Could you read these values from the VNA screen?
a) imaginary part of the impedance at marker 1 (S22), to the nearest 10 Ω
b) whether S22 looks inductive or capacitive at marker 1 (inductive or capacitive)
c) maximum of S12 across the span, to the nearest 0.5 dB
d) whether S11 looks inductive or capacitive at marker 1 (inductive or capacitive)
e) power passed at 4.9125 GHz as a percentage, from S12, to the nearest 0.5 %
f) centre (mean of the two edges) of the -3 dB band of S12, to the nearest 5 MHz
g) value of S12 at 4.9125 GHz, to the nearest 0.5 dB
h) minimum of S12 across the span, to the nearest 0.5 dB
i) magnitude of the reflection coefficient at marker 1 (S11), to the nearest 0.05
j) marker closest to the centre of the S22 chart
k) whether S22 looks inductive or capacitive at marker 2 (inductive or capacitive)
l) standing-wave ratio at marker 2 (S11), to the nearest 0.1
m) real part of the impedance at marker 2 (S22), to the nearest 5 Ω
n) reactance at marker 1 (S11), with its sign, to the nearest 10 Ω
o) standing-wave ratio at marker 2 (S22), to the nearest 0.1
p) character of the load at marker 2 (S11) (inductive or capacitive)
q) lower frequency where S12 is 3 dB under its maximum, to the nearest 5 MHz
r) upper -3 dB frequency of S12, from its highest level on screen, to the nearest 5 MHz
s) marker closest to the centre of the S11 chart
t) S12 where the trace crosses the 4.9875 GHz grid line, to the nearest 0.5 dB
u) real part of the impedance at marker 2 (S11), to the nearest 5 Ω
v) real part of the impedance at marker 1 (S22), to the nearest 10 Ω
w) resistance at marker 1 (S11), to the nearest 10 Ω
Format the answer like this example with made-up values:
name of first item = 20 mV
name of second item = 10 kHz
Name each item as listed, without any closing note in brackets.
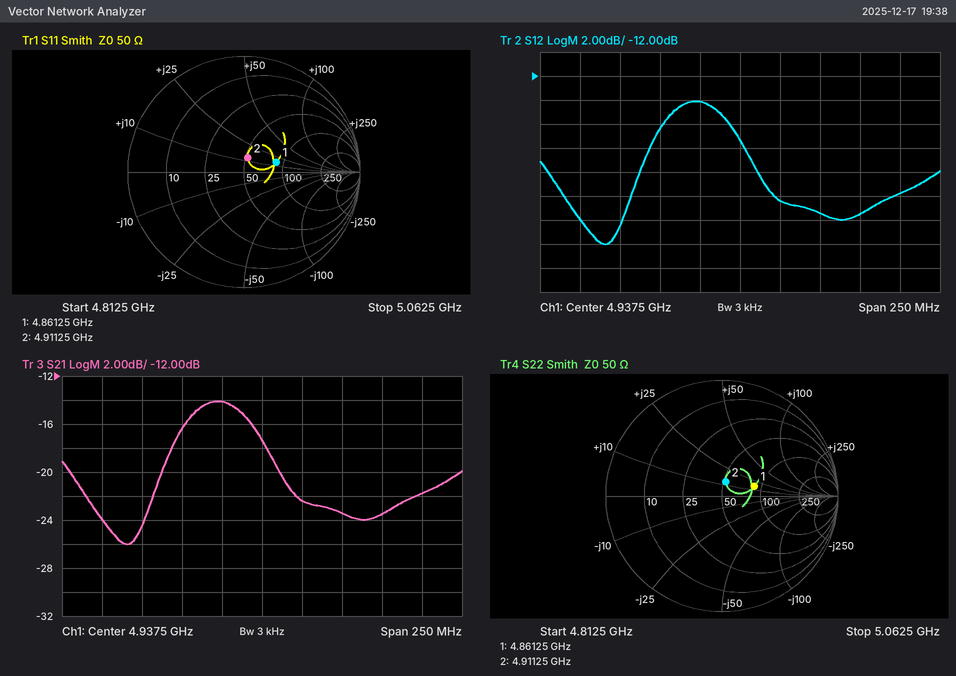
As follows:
imaginary part of the impedance at marker 1 (S22), to the nearest 10 Ω = +20 Ω
whether S22 looks inductive or capacitive at marker 1 = inductive
maximum of S12 across the span, to the nearest 0.5 dB = -14.0 dB
whether S11 looks inductive or capacitive at marker 1 = inductive
power passed at 4.9125 GHz as a percentage, from S12, to the nearest 0.5 % = 4.0 %
centre (mean of the two edges) of the -3 dB band of S12, to the nearest 5 MHz = 4.910 GHz
value of S12 at 4.9125 GHz, to the nearest 0.5 dB = -14.0 dB
minimum of S12 across the span, to the nearest 0.5 dB = -26.0 dB
magnitude of the reflection coefficient at marker 1 (S11), to the nearest 0.05 = 0.30
marker closest to the centre of the S22 chart = marker 2
whether S22 looks inductive or capacitive at marker 2 = inductive
standing-wave ratio at marker 2 (S11), to the nearest 0.1 = 1.3
real part of the impedance at marker 2 (S22), to the nearest 5 Ω = 50 Ω
reactance at marker 1 (S11), with its sign, to the nearest 10 Ω = +20 Ω
standing-wave ratio at marker 2 (S22), to the nearest 0.1 = 1.3
character of the load at marker 2 (S11) = inductive
lower frequency where S12 is 3 dB under its maximum, to the nearest 5 MHz = 4.885 GHz
upper -3 dB frequency of S12, from its highest level on screen, to the nearest 5 MHz = 4.935 GHz
marker closest to the centre of the S11 chart = marker 2
S12 where the trace crosses the 4.9875 GHz grid line, to the nearest 0.5 dB = -23.5 dB
real part of the impedance at marker 2 (S11), to the nearest 5 Ω = 50 Ω
real part of the impedance at marker 1 (S22), to the nearest 10 Ω = 90 Ω
resistance at marker 1 (S11), to the nearest 10 Ω = 90 Ω
